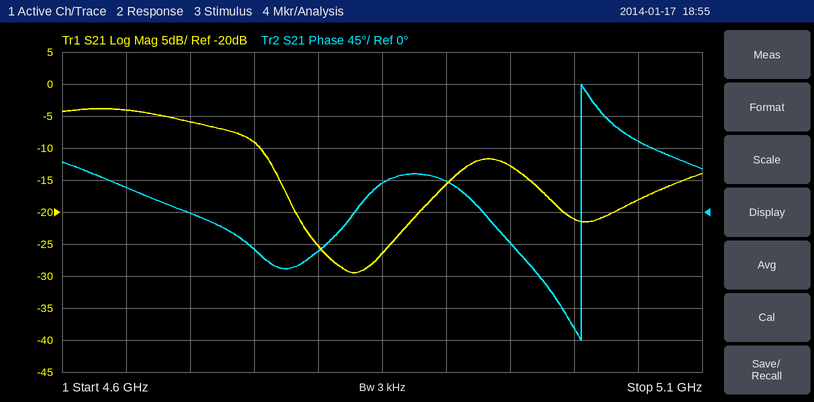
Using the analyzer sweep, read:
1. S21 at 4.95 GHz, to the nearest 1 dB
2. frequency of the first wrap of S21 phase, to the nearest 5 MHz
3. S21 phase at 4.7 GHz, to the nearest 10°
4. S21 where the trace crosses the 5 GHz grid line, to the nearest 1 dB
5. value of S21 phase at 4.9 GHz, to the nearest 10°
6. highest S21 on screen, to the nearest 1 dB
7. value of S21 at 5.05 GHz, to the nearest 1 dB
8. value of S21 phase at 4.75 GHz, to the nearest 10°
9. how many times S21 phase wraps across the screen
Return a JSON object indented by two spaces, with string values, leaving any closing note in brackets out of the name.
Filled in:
{
  "S21 at 4.95 GHz, to the nearest 1 dB": "-13 dB",
  "frequency of the first wrap of S21 phase, to the nearest 5 MHz": "5.005 GHz",
  "S21 phase at 4.7 GHz, to the nearest 10°": "0°",
  "S21 where the trace crosses the 5 GHz grid line, to the nearest 1 dB": "-21 dB",
  "value of S21 phase at 4.9 GHz, to the nearest 10°": "40°",
  "highest S21 on screen, to the nearest 1 dB": "-4 dB",
  "value of S21 at 5.05 GHz, to the nearest 1 dB": "-18 dB",
  "value of S21 phase at 4.75 GHz, to the nearest 10°": "-50°",
  "how many times S21 phase wraps across the screen": "1"
}
